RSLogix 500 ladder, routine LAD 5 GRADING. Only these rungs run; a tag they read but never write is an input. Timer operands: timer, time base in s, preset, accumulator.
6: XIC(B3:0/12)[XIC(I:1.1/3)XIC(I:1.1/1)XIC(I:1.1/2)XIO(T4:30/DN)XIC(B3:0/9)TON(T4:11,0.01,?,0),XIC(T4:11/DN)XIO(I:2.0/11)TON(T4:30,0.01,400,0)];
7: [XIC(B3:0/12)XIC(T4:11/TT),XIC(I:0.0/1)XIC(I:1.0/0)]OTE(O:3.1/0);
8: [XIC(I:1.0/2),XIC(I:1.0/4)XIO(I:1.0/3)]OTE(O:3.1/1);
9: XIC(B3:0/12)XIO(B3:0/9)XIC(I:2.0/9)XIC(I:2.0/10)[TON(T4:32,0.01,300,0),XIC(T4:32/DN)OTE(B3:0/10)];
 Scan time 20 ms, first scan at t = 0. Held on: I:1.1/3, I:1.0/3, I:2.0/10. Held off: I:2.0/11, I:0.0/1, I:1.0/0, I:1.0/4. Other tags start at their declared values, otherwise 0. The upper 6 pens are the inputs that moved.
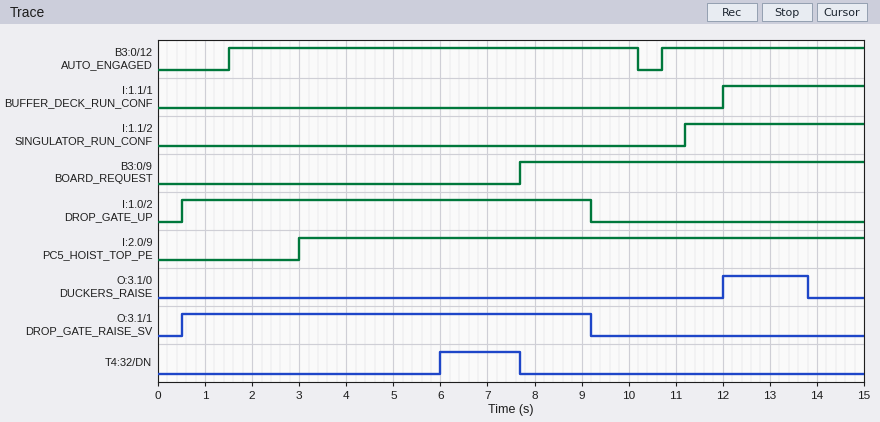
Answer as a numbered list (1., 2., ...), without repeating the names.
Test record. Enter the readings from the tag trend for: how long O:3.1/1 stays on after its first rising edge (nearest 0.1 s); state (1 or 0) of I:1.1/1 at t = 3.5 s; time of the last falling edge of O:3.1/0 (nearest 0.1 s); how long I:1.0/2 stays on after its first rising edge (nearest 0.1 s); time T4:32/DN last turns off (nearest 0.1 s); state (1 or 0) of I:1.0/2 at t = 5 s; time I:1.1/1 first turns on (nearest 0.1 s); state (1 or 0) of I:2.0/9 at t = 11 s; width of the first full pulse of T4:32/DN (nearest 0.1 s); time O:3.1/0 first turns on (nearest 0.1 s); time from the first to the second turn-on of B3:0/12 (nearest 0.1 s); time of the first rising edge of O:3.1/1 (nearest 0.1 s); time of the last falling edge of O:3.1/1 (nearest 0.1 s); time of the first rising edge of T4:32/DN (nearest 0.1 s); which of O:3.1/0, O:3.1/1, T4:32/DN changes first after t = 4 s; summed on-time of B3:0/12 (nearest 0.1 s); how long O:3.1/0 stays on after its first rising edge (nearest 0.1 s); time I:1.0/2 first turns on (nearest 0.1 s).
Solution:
1. 8.7 s
2. 0
3. 13.8 s
4. 8.7 s
5. 7.7 s
6. 1
7. 12.0 s
8. 1
9. 1.7 s
10. 12.0 s
11. 9.2 s
12. 0.5 s
13. 9.2 s
14. 6.0 s
15. T4:32/DN
16. 13.0 s
17. 1.8 s
18. 0.5 s
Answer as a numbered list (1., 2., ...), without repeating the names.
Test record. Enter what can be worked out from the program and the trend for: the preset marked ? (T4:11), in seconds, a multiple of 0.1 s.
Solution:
1. 1.8 s
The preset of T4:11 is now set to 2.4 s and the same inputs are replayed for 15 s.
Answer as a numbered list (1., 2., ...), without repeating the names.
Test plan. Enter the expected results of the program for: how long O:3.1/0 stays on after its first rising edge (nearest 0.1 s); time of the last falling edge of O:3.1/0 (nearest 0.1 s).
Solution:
1. 2.4 s
2. 14.4 s
